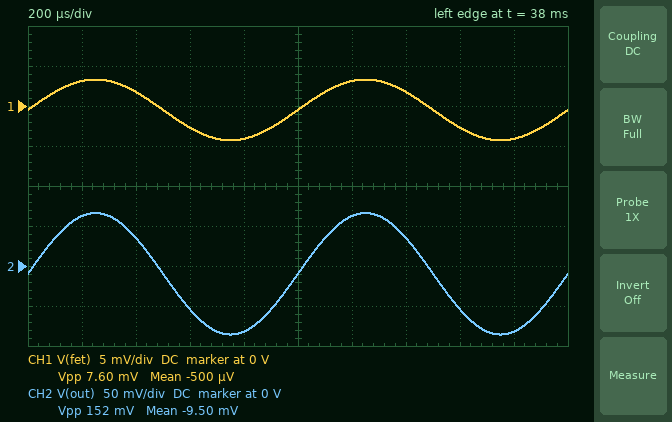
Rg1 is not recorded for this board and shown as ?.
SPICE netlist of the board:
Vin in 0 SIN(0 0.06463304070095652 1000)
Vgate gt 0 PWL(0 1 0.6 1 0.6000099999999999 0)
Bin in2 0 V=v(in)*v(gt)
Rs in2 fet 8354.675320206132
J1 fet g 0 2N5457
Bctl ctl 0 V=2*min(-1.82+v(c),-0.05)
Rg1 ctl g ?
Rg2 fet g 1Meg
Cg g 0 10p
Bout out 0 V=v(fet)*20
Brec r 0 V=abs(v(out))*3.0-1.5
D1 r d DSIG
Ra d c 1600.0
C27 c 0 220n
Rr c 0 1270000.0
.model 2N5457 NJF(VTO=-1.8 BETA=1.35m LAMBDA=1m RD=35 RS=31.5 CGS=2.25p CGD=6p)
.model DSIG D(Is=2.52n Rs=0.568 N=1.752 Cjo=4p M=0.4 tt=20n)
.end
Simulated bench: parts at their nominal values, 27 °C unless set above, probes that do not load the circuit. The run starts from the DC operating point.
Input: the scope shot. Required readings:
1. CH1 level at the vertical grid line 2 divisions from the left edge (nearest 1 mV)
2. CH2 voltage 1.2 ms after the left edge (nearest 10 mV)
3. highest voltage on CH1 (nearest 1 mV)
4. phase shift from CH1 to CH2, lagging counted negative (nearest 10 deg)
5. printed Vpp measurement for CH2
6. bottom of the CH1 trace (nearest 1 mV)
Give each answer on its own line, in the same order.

2 mV
60 mV
3 mV
0 deg
152 mV
-4 mV
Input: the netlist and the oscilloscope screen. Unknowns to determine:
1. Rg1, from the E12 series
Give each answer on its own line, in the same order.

2.7 MΩ
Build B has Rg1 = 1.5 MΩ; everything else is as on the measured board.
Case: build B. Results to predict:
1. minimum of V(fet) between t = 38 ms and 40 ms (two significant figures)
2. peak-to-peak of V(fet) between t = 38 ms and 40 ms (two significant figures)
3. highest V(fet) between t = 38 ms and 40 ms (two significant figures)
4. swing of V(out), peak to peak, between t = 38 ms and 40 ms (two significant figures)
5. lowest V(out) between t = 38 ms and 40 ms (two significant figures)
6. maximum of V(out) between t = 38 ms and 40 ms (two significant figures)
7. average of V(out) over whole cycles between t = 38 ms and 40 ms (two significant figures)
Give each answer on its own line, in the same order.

-9.3 mV
16 mV
6.3 mV
310 mV
-190 mV
130 mV
-30 mV
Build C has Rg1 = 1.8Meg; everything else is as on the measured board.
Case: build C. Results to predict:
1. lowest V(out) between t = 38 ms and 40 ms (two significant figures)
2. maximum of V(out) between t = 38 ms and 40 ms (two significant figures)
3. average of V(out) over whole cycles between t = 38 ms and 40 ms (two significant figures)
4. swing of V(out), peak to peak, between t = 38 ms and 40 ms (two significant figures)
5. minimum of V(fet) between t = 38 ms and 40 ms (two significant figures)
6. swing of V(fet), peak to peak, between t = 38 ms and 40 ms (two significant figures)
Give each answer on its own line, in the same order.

-130 mV
95 mV
-19 mV
230 mV
-6.7 mV
11 mV
